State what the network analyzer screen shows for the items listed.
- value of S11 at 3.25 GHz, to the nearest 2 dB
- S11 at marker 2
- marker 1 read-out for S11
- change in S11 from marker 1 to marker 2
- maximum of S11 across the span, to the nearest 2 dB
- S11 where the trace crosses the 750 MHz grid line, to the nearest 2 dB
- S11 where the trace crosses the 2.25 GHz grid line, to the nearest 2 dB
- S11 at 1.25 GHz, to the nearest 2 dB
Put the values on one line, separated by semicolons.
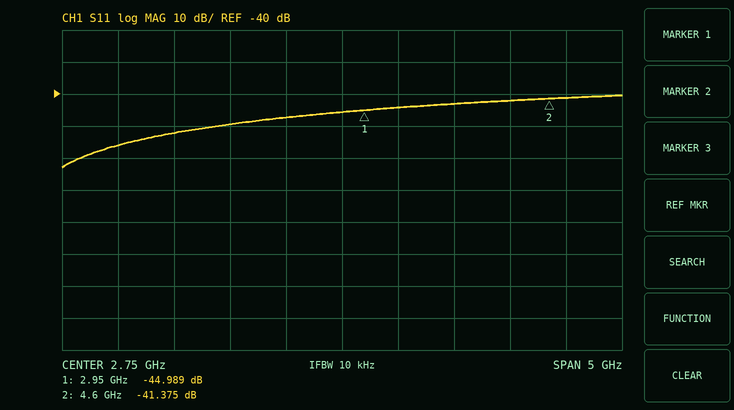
-44 dB; -41.375 dB; -44.989 dB; 3.614 dB; -40 dB; -56 dB; -48 dB; -52 dB
